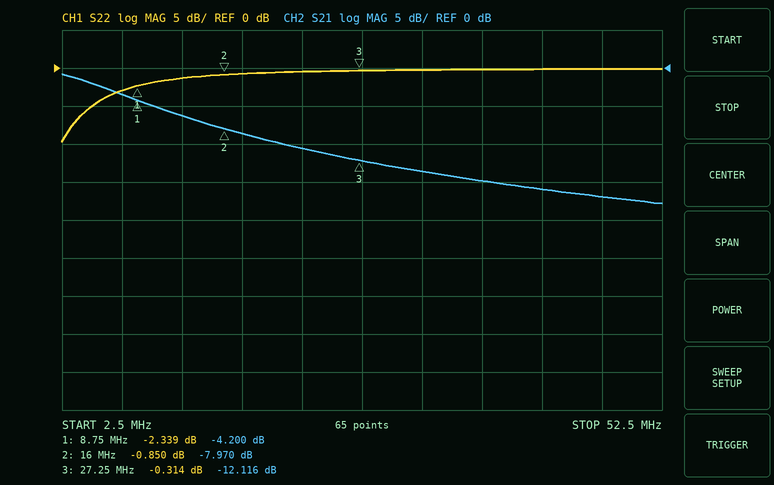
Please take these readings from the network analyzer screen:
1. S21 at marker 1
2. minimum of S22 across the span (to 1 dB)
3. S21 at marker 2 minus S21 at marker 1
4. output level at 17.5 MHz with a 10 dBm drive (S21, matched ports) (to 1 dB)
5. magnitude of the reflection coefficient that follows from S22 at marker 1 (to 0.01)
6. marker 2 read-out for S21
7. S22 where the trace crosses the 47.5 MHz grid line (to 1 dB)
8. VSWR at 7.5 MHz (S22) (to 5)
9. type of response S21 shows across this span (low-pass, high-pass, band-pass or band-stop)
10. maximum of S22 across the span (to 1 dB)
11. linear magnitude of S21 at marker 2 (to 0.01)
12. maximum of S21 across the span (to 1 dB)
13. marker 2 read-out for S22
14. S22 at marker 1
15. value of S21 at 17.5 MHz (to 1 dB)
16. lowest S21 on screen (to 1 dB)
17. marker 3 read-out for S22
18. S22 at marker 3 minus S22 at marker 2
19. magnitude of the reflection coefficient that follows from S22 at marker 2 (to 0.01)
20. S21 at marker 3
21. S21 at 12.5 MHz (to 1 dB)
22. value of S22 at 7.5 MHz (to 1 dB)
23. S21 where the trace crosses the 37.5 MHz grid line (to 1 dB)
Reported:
-4.200 dB
-10 dB
-3.770 dB
1 dBm
0.76
-7.970 dB
0 dB
5
low-pass
0 dB
0.40
-1 dB
-0.850 dB
-2.339 dB
-9 dB
-18 dB
-0.314 dB
0.536 dB
0.91
-12.116 dB
-6 dB
-3 dB
-15 dB
